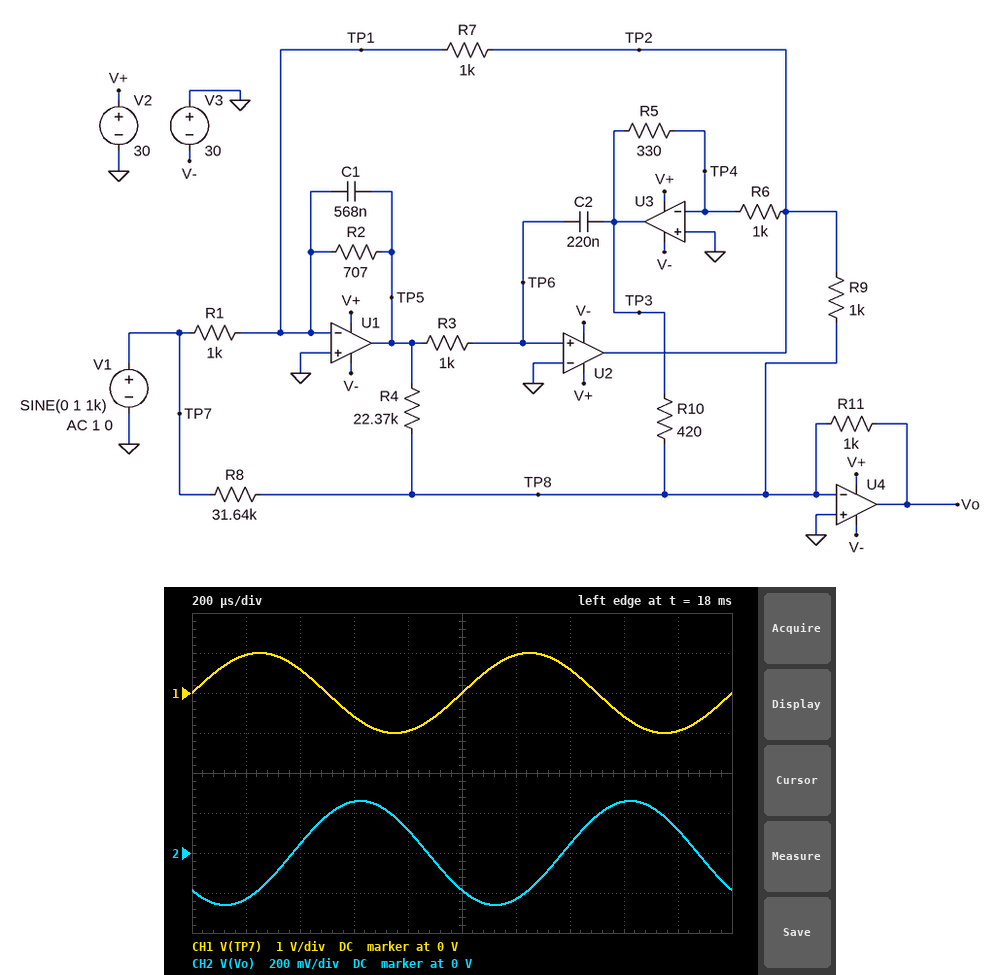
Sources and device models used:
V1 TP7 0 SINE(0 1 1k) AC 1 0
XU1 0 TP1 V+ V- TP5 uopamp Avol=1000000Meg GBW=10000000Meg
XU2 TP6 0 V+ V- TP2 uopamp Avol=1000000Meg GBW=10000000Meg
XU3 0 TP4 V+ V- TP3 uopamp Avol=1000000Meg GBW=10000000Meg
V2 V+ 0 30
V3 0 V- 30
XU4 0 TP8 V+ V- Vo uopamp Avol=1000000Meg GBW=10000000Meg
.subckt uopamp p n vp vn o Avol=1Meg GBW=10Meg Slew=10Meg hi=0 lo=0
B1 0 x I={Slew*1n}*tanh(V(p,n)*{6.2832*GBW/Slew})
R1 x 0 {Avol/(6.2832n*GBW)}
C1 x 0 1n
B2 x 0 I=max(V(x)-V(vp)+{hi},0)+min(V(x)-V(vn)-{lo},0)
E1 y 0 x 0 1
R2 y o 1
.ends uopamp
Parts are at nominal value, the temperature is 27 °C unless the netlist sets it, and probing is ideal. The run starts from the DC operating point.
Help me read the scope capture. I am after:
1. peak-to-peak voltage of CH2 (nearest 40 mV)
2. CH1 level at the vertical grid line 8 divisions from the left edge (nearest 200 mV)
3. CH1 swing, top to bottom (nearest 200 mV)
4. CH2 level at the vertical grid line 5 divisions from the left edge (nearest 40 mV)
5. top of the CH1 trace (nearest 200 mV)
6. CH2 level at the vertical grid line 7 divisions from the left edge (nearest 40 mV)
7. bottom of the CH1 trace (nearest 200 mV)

520 mV
-600 mV
2.0 V
-200 mV
1.0 V
40 mV
-1.0 V
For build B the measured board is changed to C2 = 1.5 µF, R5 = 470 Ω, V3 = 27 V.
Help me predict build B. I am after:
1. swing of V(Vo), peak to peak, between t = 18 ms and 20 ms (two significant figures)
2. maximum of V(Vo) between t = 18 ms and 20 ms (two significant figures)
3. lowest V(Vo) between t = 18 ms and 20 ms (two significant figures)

43 mV
22 mV
-22 mV
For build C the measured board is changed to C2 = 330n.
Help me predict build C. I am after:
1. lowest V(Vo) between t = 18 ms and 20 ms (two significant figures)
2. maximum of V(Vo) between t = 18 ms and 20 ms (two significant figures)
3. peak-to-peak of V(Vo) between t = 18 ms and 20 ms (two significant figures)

-150 mV
150 mV
300 mV
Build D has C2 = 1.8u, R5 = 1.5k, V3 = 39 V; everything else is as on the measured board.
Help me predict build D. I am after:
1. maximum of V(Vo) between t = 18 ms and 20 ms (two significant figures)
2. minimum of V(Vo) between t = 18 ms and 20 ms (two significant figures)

10 mV
-11 mV
